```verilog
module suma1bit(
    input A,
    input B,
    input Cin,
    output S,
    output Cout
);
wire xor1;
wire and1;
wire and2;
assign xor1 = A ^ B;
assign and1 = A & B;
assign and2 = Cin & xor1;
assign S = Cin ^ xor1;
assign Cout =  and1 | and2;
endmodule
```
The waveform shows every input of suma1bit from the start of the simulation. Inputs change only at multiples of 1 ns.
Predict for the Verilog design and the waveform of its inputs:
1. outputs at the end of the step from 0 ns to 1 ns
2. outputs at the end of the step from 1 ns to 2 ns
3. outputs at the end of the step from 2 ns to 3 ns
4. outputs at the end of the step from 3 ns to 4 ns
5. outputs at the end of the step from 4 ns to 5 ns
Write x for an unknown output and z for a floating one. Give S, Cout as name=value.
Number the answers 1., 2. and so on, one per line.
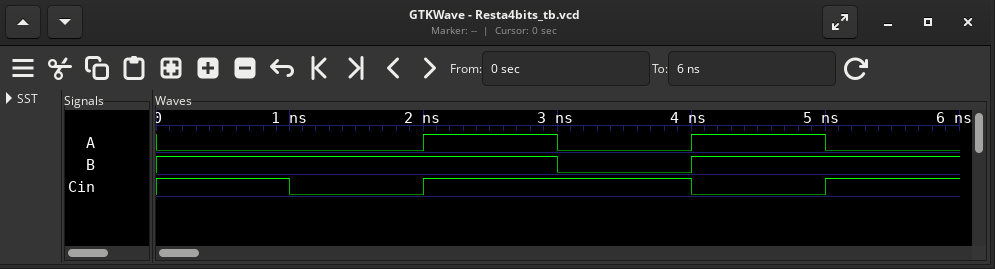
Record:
1. S=0, Cout=1
2. S=1, Cout=0
3. S=1, Cout=1
4. S=1, Cout=0
5. S=0, Cout=1
